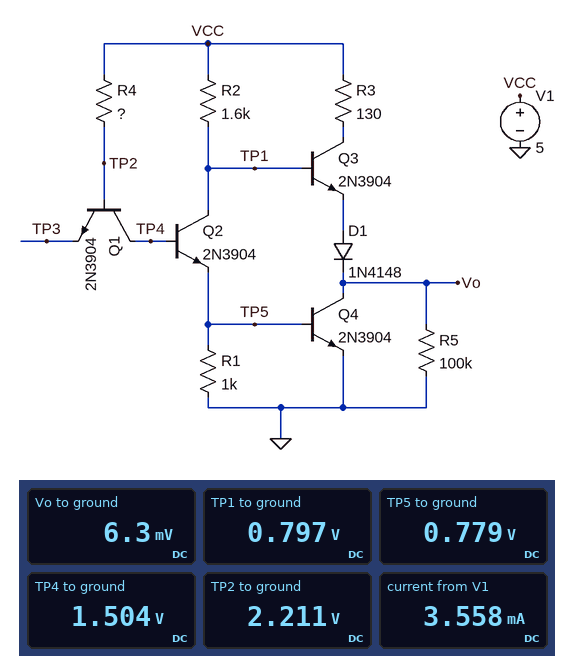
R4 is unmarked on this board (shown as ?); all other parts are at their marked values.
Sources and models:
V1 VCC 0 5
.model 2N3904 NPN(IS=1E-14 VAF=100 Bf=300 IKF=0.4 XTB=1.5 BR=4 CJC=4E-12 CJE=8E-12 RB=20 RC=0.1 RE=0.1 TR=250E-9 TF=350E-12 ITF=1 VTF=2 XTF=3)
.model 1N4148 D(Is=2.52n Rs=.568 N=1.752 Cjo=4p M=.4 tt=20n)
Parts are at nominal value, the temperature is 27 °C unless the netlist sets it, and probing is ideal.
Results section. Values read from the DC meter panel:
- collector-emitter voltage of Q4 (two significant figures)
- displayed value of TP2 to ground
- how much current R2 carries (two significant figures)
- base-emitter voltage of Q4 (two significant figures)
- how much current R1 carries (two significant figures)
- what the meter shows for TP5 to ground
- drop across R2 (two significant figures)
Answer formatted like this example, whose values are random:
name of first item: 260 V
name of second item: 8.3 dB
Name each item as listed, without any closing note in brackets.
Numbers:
collector-emitter voltage of Q4: 6.3 mV
displayed value of TP2 to ground: 2.211 V
how much current R2 carries: 2.6 mA
base-emitter voltage of Q4: 780 mV
how much current R1 carries: 780 µA
what the meter shows for TP5 to ground: 0.779 V
drop across R2: 4.2 V
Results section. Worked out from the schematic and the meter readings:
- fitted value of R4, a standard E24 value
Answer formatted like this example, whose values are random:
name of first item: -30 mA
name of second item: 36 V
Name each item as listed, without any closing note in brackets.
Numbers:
fitted value of R4, a standard E24 value: 3 kΩ
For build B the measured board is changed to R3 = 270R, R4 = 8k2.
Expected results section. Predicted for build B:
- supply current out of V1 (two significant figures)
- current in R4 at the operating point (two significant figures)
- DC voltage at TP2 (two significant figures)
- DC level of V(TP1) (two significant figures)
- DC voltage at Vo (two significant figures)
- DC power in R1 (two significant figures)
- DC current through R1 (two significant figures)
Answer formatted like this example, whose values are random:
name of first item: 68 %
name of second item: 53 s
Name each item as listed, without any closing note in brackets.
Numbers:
supply current out of V1: 3.0 mA
current in R4 at the operating point: 350 µA
DC voltage at TP2: 2.1 V
DC level of V(TP1): 790 mV
DC voltage at Vo: 6.2 mV
DC power in R1: 580 µW
DC current through R1: 760 µA
